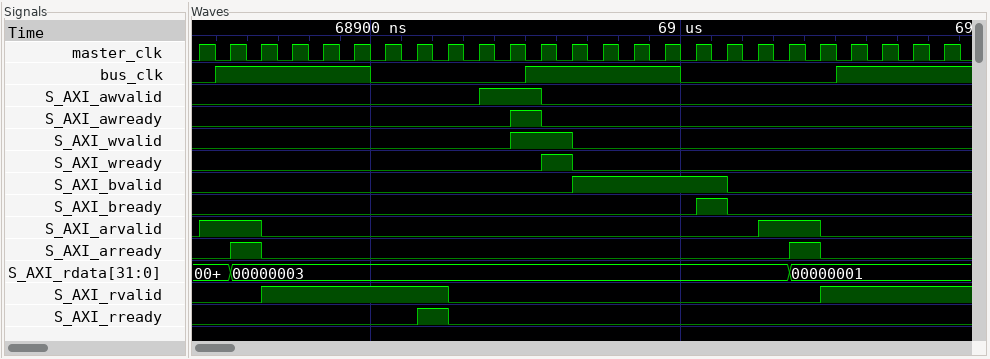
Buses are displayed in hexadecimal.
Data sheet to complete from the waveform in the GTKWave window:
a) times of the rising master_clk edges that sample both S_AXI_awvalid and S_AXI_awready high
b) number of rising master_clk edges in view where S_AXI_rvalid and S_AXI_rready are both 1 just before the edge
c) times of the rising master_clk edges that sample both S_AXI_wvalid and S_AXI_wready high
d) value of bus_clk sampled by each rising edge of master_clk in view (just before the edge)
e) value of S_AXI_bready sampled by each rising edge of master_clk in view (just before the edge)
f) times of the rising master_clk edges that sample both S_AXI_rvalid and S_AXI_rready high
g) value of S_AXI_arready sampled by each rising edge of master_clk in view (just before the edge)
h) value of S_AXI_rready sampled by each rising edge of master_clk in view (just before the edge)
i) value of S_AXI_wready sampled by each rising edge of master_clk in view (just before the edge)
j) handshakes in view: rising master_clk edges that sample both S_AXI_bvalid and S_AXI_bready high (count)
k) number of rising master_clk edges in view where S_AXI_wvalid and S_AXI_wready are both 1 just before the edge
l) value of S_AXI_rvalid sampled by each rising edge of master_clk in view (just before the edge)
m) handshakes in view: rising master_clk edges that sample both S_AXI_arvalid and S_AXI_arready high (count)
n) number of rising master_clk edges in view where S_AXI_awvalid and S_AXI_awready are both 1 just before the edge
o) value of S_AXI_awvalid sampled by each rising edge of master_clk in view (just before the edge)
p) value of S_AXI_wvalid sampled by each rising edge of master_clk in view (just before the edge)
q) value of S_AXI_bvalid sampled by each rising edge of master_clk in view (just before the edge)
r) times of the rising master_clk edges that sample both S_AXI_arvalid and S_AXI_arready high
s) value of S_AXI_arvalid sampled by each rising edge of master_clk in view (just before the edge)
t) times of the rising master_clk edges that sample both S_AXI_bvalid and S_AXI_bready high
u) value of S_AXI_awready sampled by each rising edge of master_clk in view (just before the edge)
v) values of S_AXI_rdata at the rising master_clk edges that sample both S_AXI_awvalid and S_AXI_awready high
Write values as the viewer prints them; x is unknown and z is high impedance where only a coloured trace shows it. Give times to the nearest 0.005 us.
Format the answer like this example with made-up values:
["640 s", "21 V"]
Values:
["68.955 us", "1", "68.965 us", "0 1 1 1 1 1 0 0 0 0 0 1 1 1 1 1 0 0 0 0 0 1 1 1 1", "0 0 0 0 0 0 0 0 0 0 0 0 0 0 0 0 0 1 0 0 0 0 0 0 0", "68.925 us", "0 0 1 0 0 0 0 0 0 0 0 0 0 0 0 0 0 0 0 0 1 0 0 0 0", "0 0 0 0 0 0 0 0 1 0 0 0 0 0 0 0 0 0 0 0 0 0 0 0 0", "0 0 0 0 0 0 0 0 0 0 0 0 1 0 0 0 0 0 0 0 0 0 0 0 0", "1", "1", "0 0 0 1 1 1 1 1 1 0 0 0 0 0 0 0 0 0 0 0 0 1 1 1 1", "2", "1", "0 0 0 0 0 0 0 0 0 0 1 1 0 0 0 0 0 0 0 0 0 0 0 0 0", "0 0 0 0 0 0 0 0 0 0 0 1 1 0 0 0 0 0 0 0 0 0 0 0 0", "0 0 0 0 0 0 0 0 0 0 0 0 0 1 1 1 1 1 0 0 0 0 0 0 0", "68.865 us, 69.045 us", "0 1 1 0 0 0 0 0 0 0 0 0 0 0 0 0 0 0 0 1 1 0 0 0 0", "69.015 us", "0 0 0 0 0 0 0 0 0 0 0 1 0 0 0 0 0 0 0 0 0 0 0 0 0", "00000003"]
